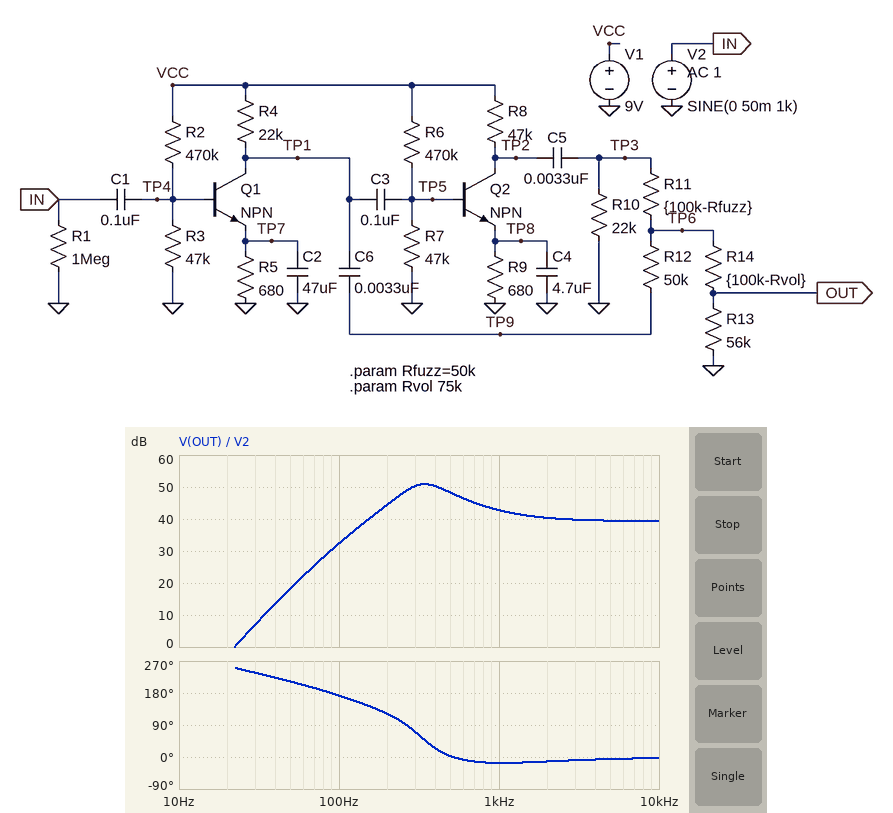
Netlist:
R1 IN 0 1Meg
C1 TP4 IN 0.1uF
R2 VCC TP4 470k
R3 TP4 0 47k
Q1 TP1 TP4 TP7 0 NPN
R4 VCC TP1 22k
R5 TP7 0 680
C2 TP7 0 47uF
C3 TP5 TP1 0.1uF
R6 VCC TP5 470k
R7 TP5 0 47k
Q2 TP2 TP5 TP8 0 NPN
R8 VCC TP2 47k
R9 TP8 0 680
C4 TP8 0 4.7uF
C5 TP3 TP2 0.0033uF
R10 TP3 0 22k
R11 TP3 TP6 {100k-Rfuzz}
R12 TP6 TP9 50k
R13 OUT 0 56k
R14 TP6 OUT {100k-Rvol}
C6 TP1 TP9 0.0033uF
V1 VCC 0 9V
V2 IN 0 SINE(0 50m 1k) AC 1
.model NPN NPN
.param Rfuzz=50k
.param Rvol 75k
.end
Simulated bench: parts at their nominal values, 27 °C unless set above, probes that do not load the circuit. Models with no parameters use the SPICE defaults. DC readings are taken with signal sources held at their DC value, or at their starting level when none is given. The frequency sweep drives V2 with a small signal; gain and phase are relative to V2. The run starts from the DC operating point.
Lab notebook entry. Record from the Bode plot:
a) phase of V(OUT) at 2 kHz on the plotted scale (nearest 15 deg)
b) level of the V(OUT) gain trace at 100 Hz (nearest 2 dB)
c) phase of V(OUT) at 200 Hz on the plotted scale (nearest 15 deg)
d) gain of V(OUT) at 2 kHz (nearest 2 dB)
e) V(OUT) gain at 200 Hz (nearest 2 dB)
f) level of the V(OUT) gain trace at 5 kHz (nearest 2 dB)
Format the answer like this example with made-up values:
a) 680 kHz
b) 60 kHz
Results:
a) -15 deg
b) 32 dB
c) 120 deg
d) 40 dB
e) 44 dB
f) 40 dB
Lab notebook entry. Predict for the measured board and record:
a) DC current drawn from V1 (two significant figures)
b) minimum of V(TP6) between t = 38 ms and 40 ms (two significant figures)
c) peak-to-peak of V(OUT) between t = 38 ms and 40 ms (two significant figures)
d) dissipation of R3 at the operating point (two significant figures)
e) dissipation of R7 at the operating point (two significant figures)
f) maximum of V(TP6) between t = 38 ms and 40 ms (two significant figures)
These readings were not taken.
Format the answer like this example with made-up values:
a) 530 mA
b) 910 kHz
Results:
a) 220 µA
b) -1.3 V
c) 1.5 V
d) 13 µW
e) 13 µW
f) 870 mV
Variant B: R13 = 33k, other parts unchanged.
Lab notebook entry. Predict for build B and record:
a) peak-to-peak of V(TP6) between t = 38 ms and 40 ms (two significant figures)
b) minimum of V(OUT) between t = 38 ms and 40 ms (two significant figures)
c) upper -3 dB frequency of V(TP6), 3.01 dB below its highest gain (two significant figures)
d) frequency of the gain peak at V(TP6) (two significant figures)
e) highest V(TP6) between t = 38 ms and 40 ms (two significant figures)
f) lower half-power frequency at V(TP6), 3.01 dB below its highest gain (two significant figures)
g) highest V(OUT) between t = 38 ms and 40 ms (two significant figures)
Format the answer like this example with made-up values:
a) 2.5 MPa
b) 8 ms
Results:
a) 2.0 V
b) -700 mV
c) 570 Hz
d) 370 Hz
e) 790 mV
f) 260 Hz
g) 450 mV
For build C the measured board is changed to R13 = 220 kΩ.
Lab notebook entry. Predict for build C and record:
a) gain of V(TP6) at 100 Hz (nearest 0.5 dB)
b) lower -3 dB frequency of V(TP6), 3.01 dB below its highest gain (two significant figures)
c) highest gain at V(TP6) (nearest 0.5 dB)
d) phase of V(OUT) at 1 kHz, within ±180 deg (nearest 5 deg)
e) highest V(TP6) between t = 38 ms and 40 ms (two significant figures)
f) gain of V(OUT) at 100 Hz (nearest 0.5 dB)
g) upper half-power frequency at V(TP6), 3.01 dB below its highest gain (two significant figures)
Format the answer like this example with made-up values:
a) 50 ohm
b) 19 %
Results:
a) 39.0 dB
b) 220 Hz
c) 56.5 dB
d) -20 deg
e) 1.1 V
f) 38.0 dB
g) 420 Hz
